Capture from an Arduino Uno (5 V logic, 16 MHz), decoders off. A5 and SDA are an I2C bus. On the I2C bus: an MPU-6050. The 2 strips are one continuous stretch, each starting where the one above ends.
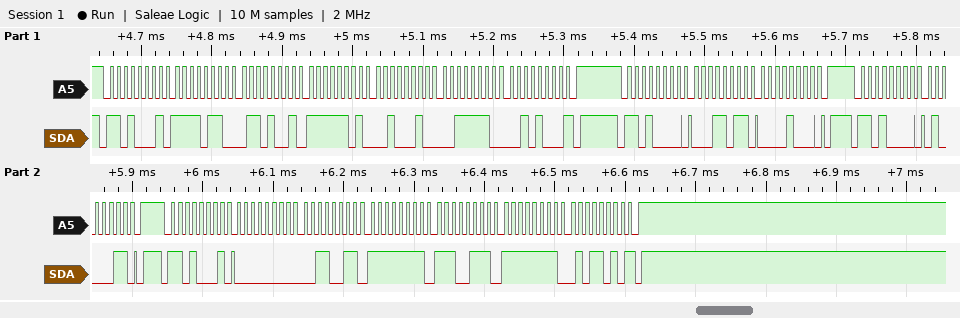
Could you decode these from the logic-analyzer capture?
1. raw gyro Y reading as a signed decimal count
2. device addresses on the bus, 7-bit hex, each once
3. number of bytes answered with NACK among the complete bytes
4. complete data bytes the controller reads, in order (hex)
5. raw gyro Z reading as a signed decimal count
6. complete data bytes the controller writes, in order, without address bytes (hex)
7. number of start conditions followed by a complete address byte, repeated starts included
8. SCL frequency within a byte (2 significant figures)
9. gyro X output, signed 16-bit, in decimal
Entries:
-25
0x68
2
F6 69 FD 22 3E 28 00 33 FF E7 FF 5A
-166
1B 08 43
4
100 kHz
51
